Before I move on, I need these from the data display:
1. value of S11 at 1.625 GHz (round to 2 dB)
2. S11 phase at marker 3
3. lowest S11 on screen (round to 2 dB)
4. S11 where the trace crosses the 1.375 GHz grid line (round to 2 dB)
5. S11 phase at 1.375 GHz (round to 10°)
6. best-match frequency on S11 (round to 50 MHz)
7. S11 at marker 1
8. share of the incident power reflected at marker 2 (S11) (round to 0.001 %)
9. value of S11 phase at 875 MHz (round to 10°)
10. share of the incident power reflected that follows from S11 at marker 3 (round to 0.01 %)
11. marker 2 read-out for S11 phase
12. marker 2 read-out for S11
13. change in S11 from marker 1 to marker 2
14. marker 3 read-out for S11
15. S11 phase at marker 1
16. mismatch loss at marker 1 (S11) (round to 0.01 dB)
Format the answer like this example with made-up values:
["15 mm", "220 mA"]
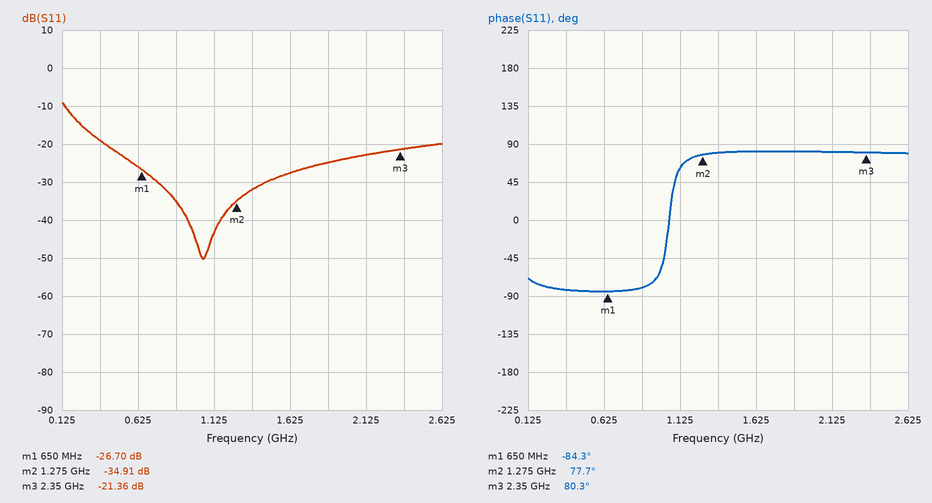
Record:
["-28 dB", "80.3°", "-50 dB", "-32 dB", "80°", "1.05 GHz", "-26.70 dB", "0.032 %", "-80°", "0.73 %", "77.7°", "-34.91 dB", "-8.21 dB", "-21.36 dB", "-84.3°", "0.01 dB"]
